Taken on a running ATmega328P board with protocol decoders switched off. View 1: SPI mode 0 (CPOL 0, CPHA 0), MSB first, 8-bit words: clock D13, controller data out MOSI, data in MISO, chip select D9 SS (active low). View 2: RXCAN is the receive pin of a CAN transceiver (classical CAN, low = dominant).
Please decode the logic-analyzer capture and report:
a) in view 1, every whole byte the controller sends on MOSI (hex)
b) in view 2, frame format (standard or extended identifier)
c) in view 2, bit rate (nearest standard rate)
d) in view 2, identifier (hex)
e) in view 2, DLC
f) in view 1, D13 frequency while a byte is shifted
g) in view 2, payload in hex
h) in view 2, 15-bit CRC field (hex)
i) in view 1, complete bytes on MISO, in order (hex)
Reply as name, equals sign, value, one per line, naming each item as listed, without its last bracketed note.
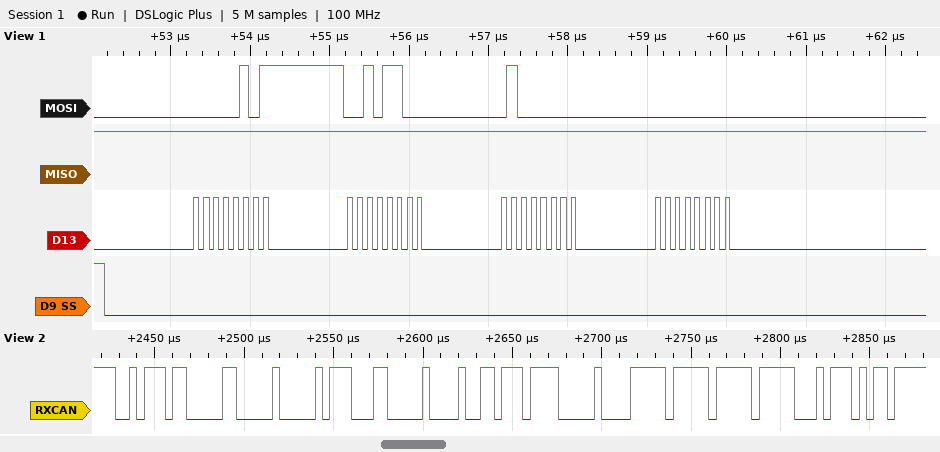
in view 1, every whole byte the controller sends on MOSI = 05 2C 40 00
in view 2, frame format = standard
in view 2, bit rate = 250 kbit/s
in view 2, identifier = 0x2EC
in view 2, DLC = 8
in view 1, D13 frequency while a byte is shifted = 8 MHz
in view 2, payload in hex = 00 E3 00 4D DE 00 FF FF
in view 2, 15-bit CRC field = 0x7975
in view 1, complete bytes on MISO, in order = FF FF FF FF
